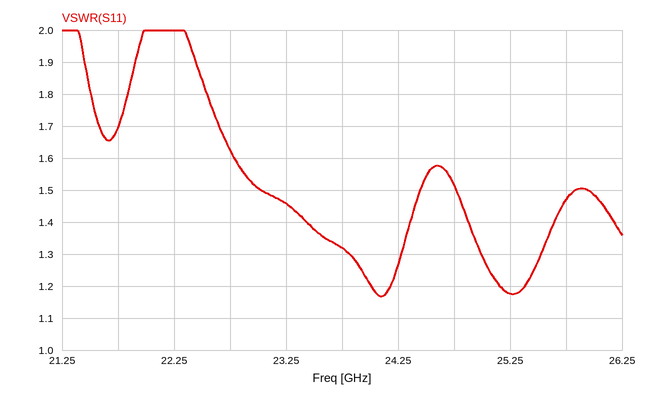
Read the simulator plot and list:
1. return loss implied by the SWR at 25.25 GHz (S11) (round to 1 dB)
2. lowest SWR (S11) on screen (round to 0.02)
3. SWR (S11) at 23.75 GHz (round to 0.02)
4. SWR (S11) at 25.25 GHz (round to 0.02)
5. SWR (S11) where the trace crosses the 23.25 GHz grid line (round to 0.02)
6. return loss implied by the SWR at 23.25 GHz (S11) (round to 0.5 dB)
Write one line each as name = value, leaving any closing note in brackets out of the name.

return loss implied by the SWR at 25.25 GHz (S11) = 22 dB
lowest SWR (S11) on screen = 1.16
SWR (S11) at 23.75 GHz = 1.32
SWR (S11) at 25.25 GHz = 1.18
SWR (S11) where the trace crosses the 23.25 GHz grid line = 1.46
return loss implied by the SWR at 23.25 GHz (S11) = 14.5 dB
